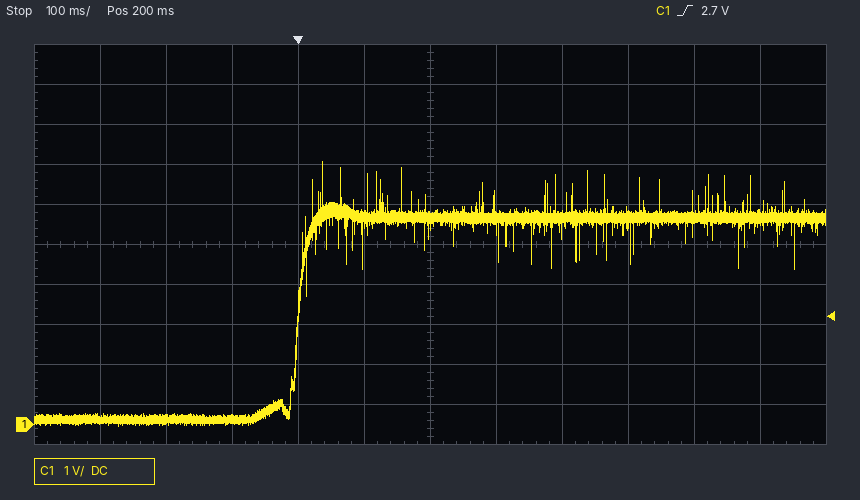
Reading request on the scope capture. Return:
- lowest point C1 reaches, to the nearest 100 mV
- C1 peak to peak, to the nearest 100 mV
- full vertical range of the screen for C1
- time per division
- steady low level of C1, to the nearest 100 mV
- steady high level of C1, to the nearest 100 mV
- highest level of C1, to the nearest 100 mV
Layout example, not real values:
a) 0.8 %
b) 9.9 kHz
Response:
a) 0.0 V
b) 6.6 V
c) 10 V
d) 100 ms
e) 100 mV
f) 5.2 V
g) 6.6 V
